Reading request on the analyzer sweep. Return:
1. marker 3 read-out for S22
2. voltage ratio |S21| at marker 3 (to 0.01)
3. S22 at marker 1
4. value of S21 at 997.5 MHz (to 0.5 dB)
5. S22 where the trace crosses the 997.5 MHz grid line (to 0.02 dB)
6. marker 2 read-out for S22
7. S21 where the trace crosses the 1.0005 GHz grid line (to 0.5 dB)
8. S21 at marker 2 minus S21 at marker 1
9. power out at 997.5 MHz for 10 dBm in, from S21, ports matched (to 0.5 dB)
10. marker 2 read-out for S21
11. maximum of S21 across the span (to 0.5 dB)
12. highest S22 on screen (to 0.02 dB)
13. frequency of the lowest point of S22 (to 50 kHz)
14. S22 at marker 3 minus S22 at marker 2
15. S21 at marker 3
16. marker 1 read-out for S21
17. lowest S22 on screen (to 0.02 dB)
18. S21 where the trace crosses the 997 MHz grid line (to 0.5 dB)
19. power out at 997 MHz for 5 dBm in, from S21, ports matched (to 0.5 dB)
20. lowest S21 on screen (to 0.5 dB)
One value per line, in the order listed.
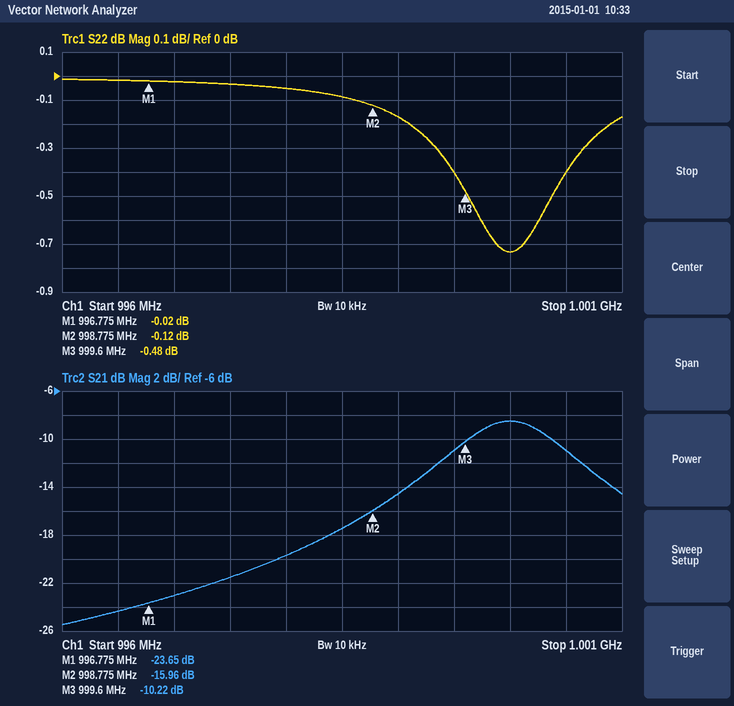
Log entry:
-0.48 dB
0.31
-0.02 dB
-21.5 dB
-0.04 dB
-0.12 dB
-11.0 dB
7.69 dB
-11.5 dBm
-15.96 dB
-8.5 dB
-0.02 dB
1.00000 GHz
-0.36 dB
-10.22 dB
-23.65 dB
-0.74 dB
-23.0 dB
-18.0 dBm
-25.5 dB
